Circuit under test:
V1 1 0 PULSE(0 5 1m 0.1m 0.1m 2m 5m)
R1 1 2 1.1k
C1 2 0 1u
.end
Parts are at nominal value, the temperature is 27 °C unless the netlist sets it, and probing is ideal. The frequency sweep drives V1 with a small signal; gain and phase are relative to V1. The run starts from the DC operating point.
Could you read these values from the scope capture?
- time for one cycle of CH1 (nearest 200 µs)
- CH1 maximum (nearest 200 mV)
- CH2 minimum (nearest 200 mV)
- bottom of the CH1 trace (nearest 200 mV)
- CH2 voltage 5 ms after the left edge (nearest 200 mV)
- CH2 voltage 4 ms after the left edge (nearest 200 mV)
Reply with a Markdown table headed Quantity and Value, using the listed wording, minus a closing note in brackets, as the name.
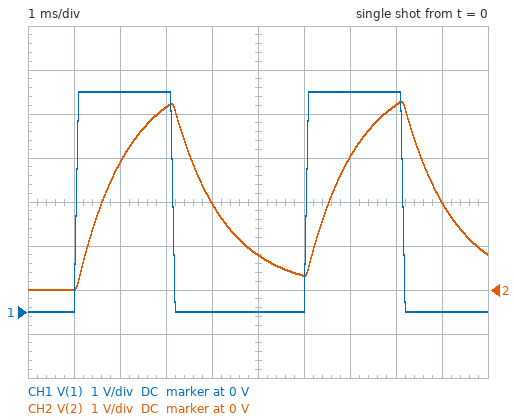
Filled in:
| Quantity | Value |
|---|---|
| time for one cycle of CH1 | 5.0 ms |
| CH1 maximum | 5.0 V |
| CH2 minimum | 0 V |
| bottom of the CH1 trace | 0 V |
| CH2 voltage 5 ms after the left edge | 800 mV |
| CH2 voltage 4 ms after the left edge | 2.0 V |
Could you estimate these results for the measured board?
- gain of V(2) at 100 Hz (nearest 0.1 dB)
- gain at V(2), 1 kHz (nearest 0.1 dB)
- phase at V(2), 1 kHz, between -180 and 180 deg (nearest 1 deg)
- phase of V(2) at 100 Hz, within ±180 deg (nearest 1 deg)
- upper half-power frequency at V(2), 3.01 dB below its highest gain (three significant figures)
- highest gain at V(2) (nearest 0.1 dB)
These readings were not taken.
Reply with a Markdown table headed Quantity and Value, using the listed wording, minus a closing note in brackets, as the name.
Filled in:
| Quantity | Value |
|---|---|
| gain of V(2) at 100 Hz | -1.7 dB |
| gain at V(2), 1 kHz | -16.9 dB |
| phase at V(2), 1 kHz, between -180 and 180 deg | -82 deg |
| phase of V(2) at 100 Hz, within ±180 deg | -35 deg |
| upper half-power frequency at V(2), 3.01 dB below its highest gain | 145 Hz |
| highest gain at V(2) | 0 dB |
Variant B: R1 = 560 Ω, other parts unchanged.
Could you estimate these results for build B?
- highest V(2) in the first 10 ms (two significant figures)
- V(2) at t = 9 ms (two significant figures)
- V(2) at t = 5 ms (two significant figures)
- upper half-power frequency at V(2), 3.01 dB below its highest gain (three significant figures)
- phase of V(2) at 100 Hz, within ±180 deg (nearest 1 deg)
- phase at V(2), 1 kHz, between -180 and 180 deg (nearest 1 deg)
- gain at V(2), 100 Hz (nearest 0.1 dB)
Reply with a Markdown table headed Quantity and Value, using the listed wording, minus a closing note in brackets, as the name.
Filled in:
| Quantity | Value |
|---|---|
| highest V(2) in the first 10 ms | 4.9 V |
| V(2) at t = 9 ms | 1.1 V |
| V(2) at t = 5 ms | 180 mV |
| upper half-power frequency at V(2), 3.01 dB below its highest gain | 284 Hz |
| phase of V(2) at 100 Hz, within ±180 deg | -19 deg |
| phase at V(2), 1 kHz, between -180 and 180 deg | -74 deg |
| gain at V(2), 100 Hz | -0.5 dB |
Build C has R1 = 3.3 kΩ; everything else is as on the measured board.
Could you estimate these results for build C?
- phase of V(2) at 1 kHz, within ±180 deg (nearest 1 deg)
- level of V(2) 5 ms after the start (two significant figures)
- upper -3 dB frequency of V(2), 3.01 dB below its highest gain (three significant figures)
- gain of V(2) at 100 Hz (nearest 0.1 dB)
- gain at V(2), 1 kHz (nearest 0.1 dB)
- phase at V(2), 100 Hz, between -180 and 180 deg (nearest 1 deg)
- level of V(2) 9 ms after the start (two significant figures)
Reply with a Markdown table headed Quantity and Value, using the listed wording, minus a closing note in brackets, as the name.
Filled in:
| Quantity | Value |
|---|---|
| phase of V(2) at 1 kHz, within ±180 deg | -87 deg |
| level of V(2) 5 ms after the start | 1.3 V |
| upper -3 dB frequency of V(2), 3.01 dB below its highest gain | 48.2 Hz |
| gain of V(2) at 100 Hz | -7.2 dB |
| gain at V(2), 1 kHz | -26.3 dB |
| phase at V(2), 100 Hz, between -180 and 180 deg | -64 deg |
| level of V(2) 9 ms after the start | 2.2 V |
